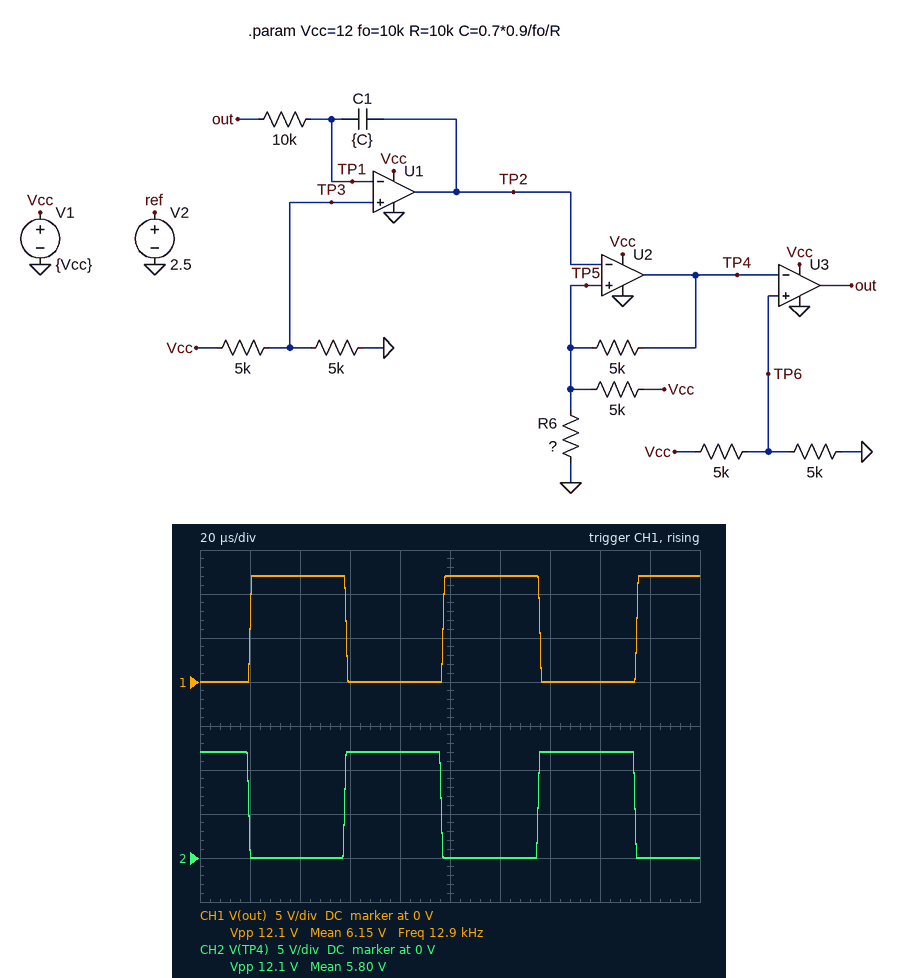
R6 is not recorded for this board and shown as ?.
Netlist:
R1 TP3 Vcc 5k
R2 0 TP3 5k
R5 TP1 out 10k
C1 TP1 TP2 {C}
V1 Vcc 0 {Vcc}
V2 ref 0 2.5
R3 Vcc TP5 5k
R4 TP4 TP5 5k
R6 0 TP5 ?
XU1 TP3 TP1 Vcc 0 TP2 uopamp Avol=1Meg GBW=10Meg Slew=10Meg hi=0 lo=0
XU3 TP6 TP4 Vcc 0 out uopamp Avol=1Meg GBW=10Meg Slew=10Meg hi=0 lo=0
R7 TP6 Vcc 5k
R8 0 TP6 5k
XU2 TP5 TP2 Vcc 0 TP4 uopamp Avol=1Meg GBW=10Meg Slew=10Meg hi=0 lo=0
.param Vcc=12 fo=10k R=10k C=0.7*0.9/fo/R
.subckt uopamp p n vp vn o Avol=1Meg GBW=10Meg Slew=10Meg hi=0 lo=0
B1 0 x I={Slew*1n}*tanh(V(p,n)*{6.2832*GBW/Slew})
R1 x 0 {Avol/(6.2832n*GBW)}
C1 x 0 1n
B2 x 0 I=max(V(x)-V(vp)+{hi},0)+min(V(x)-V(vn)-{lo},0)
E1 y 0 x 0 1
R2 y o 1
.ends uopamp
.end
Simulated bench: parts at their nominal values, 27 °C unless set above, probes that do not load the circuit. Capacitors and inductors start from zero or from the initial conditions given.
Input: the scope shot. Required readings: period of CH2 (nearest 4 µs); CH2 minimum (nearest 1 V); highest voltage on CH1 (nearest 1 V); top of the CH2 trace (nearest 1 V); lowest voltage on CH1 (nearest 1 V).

76 µs
0 V
12 V
12 V
0 V
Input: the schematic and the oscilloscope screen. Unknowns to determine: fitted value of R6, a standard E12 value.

3.3 kΩ
